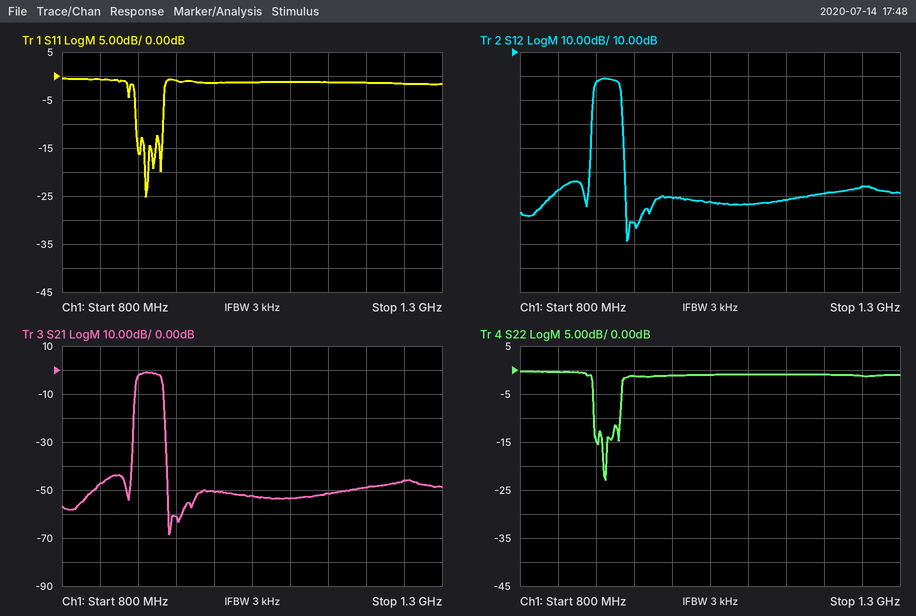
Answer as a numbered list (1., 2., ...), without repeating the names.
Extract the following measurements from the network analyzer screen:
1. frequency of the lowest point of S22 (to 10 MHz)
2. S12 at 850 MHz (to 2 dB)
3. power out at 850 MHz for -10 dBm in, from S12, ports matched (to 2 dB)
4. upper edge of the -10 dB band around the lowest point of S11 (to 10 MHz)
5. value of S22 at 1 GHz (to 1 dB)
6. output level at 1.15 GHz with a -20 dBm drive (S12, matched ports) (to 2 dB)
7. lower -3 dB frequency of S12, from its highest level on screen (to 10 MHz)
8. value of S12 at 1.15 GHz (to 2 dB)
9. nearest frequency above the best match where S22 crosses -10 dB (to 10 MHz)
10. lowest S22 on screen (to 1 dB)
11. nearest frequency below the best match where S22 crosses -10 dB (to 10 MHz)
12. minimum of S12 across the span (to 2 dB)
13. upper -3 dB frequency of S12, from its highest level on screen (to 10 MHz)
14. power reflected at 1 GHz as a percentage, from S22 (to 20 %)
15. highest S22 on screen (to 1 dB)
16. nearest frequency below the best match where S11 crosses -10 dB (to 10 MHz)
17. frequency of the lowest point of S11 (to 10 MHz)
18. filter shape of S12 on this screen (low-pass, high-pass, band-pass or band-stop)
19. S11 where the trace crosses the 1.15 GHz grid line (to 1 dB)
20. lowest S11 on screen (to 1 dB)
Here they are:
1. 910 MHz
2. -48 dB
3. -58 dBm
4. 930 MHz
5. -1 dB
6. -72 dBm
7. 900 MHz
8. -52 dB
9. 930 MHz
10. -23 dB
11. 900 MHz
12. -68 dB
13. 930 MHz
14. 80 %
15. 0 dB
16. 900 MHz
17. 910 MHz
18. band-pass
19. -1 dB
20. -25 dB
